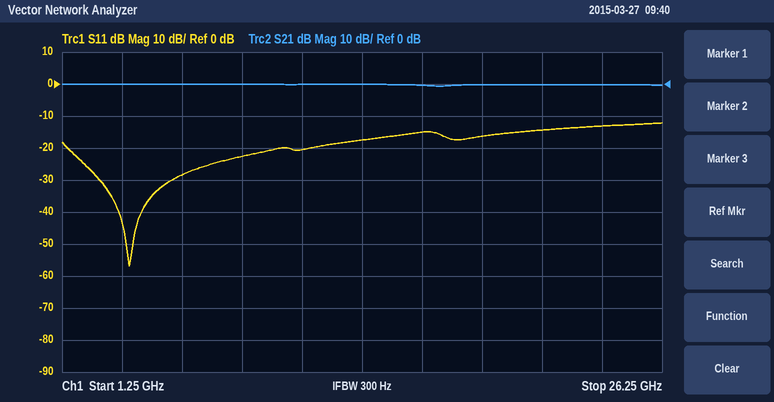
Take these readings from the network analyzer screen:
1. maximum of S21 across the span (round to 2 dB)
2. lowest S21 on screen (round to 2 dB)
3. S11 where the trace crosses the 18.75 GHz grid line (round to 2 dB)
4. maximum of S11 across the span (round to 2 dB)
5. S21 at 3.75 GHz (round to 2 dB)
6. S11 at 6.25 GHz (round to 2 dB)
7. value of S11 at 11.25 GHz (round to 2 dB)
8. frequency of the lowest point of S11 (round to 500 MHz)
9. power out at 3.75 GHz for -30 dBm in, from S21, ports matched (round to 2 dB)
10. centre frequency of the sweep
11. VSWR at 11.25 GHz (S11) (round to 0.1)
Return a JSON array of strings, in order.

["0 dB", "0 dB", "-16 dB", "-12 dB", "0 dB", "-28 dB", "-20 dB", "4.0 GHz", "-30 dBm", "13.75 GHz", "1.2"]
